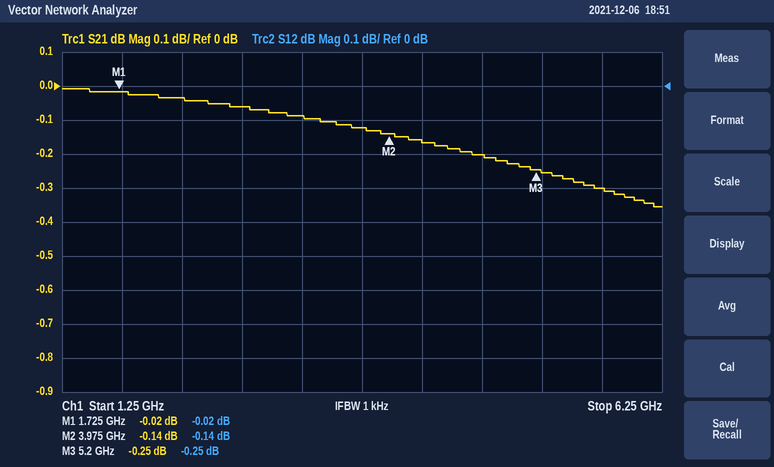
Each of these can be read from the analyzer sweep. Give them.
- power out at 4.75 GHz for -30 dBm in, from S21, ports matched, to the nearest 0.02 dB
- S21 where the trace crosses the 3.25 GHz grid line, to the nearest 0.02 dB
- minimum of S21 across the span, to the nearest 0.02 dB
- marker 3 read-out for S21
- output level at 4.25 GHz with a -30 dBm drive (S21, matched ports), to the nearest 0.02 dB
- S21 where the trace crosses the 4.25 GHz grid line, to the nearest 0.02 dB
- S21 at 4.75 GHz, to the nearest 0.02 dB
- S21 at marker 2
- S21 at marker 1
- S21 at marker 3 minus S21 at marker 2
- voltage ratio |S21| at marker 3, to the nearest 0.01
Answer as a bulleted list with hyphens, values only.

- -30.20 dBm
- -0.08 dB
- -0.36 dB
- -0.25 dB
- -30.16 dBm
- -0.16 dB
- -0.20 dB
- -0.14 dB
- -0.02 dB
- -0.11 dB
- 0.97
